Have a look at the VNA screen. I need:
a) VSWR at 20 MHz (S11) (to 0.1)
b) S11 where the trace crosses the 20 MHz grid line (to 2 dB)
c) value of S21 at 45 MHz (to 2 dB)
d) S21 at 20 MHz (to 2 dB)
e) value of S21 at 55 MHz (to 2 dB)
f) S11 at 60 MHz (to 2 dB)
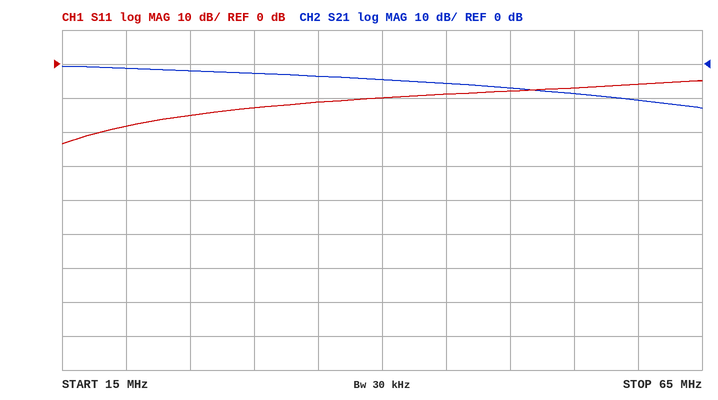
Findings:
1.3
-18 dB
-6 dB
-2 dB
-8 dB
-6 dB
